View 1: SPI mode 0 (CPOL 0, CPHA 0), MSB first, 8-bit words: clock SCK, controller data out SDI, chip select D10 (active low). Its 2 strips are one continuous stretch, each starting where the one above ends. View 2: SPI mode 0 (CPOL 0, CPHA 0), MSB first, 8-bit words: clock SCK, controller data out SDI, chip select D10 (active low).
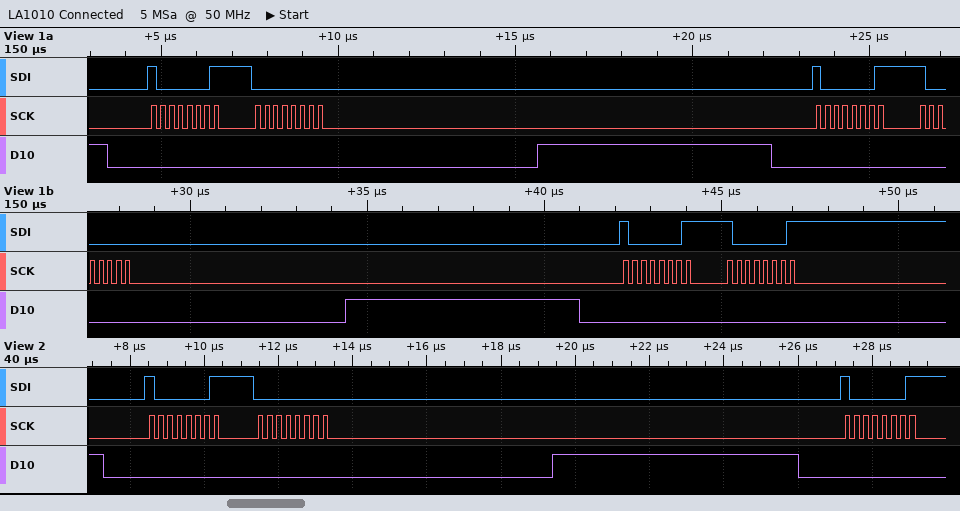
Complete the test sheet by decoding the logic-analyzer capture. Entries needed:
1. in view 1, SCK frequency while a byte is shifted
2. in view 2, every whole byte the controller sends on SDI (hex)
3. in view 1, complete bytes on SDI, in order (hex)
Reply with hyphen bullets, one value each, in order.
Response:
- 4 MHz
- 81 00 81
- 81 00 81 80 81 81
